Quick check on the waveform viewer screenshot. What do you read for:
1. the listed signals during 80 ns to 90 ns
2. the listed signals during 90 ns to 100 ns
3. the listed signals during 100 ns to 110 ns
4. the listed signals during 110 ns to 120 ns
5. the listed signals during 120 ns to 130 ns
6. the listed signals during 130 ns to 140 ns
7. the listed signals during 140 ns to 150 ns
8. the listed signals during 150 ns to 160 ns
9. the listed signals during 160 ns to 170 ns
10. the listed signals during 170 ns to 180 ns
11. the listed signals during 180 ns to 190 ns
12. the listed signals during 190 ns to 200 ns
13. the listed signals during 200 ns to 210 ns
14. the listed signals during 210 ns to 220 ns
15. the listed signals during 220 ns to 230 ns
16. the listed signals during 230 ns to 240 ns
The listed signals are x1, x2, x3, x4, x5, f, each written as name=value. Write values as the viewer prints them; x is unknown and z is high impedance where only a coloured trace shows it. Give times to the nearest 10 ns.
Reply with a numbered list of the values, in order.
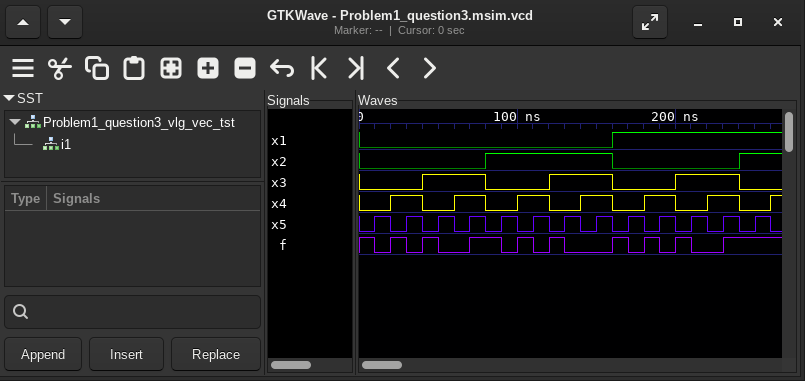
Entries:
1. x1=0, x2=1, x3=0, x4=0, x5=0, f=1
2. x1=0, x2=1, x3=0, x4=0, x5=1, f=0
3. x1=0, x2=1, x3=0, x4=1, x5=0, f=1
4. x1=0, x2=1, x3=0, x4=1, x5=1, f=0
5. x1=0, x2=1, x3=1, x4=0, x5=0, f=1
6. x1=0, x2=1, x3=1, x4=0, x5=1, f=0
7. x1=0, x2=1, x3=1, x4=1, x5=0, f=0
8. x1=0, x2=1, x3=1, x4=1, x5=1, f=0
9. x1=1, x2=0, x3=0, x4=0, x5=0, f=1
10. x1=1, x2=0, x3=0, x4=0, x5=1, f=0
11. x1=1, x2=0, x3=0, x4=1, x5=0, f=1
12. x1=1, x2=0, x3=0, x4=1, x5=1, f=0
13. x1=1, x2=0, x3=1, x4=0, x5=0, f=1
14. x1=1, x2=0, x3=1, x4=0, x5=1, f=0
15. x1=1, x2=0, x3=1, x4=1, x5=0, f=0
16. x1=1, x2=0, x3=1, x4=1, x5=1, f=1
